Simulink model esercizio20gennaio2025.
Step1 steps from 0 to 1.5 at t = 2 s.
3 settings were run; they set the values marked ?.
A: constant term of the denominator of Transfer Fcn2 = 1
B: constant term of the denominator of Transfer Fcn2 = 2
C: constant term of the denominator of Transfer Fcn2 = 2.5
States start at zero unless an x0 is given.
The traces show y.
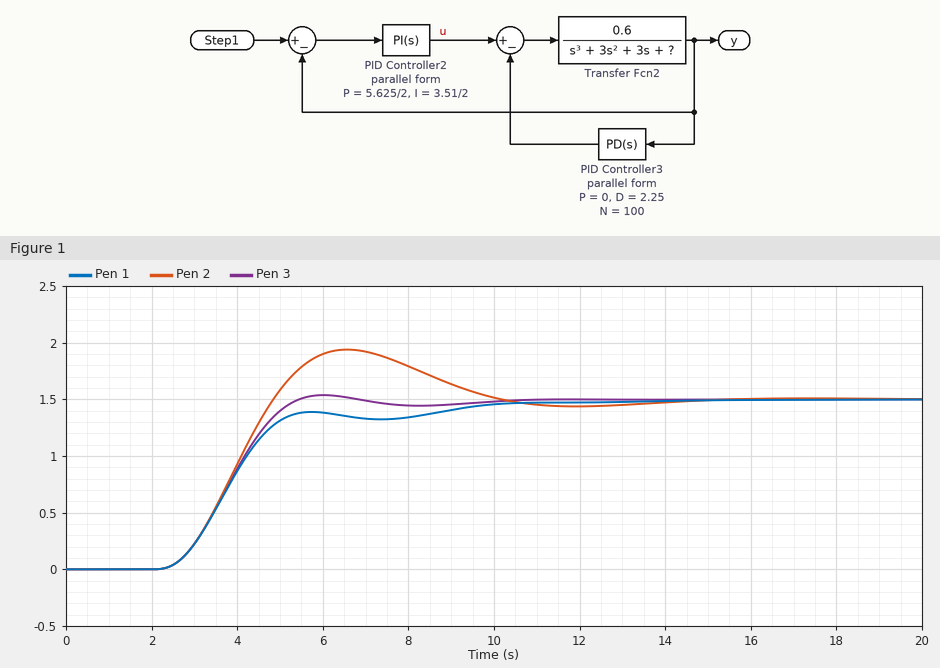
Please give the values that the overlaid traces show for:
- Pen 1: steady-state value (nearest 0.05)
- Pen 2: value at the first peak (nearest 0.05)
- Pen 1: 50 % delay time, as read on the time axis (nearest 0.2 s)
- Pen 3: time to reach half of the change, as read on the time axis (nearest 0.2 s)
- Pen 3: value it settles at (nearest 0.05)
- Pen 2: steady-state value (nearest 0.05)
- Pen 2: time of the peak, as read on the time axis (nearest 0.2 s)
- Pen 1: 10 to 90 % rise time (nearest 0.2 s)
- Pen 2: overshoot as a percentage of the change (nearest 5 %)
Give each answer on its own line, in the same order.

1.50
1.95
3.8 s
3.8 s
1.50
1.50
6.6 s
2.4 s
30 %
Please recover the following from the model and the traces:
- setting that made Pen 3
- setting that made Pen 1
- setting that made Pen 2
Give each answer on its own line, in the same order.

B
C
A
